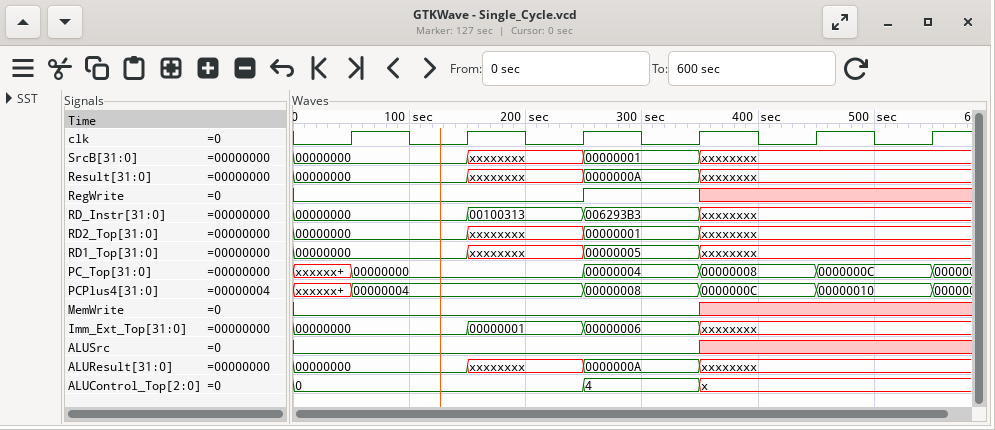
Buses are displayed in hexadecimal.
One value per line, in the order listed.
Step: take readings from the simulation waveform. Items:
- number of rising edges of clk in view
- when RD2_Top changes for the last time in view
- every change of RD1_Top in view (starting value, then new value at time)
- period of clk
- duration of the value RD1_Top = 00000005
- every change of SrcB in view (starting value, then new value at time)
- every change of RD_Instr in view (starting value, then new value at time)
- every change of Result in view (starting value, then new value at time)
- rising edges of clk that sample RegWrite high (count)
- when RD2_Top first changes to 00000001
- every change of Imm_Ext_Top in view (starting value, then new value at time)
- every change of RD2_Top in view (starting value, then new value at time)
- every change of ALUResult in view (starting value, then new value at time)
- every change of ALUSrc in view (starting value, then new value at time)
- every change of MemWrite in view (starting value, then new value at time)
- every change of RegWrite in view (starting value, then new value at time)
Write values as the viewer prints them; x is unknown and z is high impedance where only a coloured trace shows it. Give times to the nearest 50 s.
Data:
6
350 s
00000000, xxxxxxxx at 150 s, 00000005 at 250 s, xxxxxxxx at 350 s
100 s
100 s
00000000, xxxxxxxx at 150 s, 00000001 at 250 s, xxxxxxxx at 350 s
00000000, 00100313 at 150 s, 006293B3 at 250 s, xxxxxxxx at 350 s
00000000, xxxxxxxx at 150 s, 0000000A at 250 s, xxxxxxxx at 350 s
1
250 s
00000000, 00000001 at 150 s, 00000006 at 250 s, xxxxxxxx at 350 s
00000000, xxxxxxxx at 150 s, 00000001 at 250 s, xxxxxxxx at 350 s
00000000, xxxxxxxx at 150 s, 0000000A at 250 s, xxxxxxxx at 350 s
0, x at 350 s
0, x at 350 s
0, 1 at 250 s, x at 350 s
